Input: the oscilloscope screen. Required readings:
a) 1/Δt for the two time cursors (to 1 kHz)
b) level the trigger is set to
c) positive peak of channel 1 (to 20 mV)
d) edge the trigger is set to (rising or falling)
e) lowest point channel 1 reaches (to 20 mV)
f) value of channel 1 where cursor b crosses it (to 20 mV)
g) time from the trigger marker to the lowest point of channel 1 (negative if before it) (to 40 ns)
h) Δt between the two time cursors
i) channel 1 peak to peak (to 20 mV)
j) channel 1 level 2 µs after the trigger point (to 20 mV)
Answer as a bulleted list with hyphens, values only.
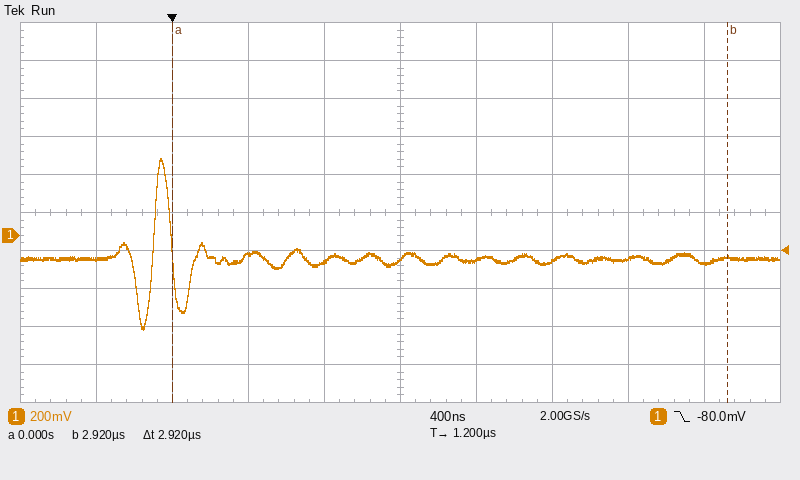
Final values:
- 342 kHz
- -80.0 mV
- 400 mV
- falling
- -500 mV
- -120 mV
- -160 ns
- 2.92 µs
- 900 mV
- -140 mV
